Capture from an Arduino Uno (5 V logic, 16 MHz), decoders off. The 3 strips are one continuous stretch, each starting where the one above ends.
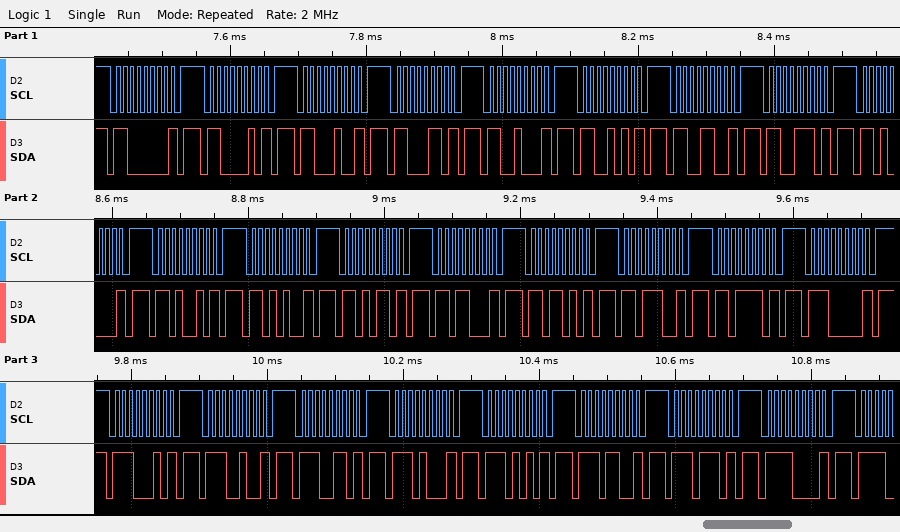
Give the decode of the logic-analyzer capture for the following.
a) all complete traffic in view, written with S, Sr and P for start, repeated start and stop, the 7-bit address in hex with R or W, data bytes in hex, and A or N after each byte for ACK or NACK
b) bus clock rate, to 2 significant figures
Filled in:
S 60W N P S 61W N P S 62W N P S 63W N P S 64W N P S 65W N P S 66W N P S 67W N P S 68W N P S 69W N P S 6AW N P S 6BW N P S 6CW N P S 6DW N P S 6EW N P S 6FW N P S 70W N P S 71W N P S 72W N P S 73W N P S 74W N P S 75W N P S 76W N P S 77W N P S 78W N P
100 kHz
